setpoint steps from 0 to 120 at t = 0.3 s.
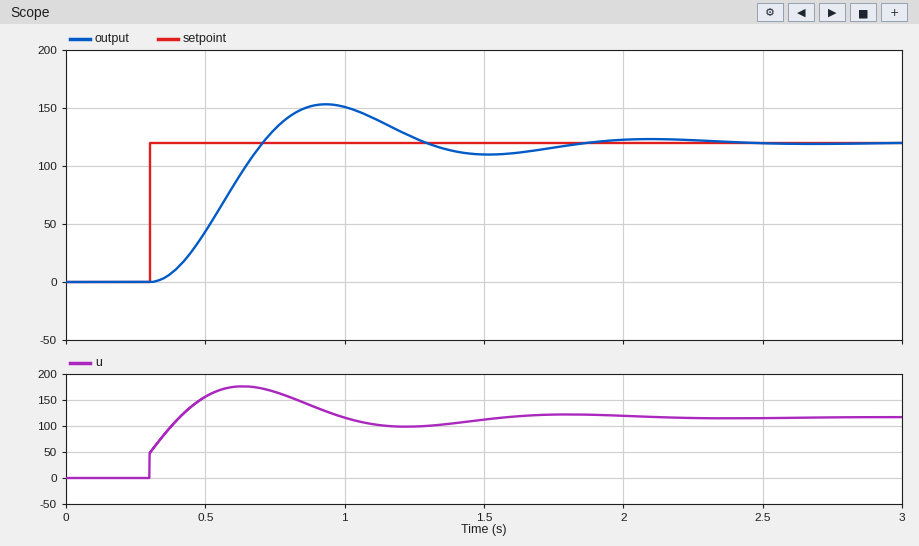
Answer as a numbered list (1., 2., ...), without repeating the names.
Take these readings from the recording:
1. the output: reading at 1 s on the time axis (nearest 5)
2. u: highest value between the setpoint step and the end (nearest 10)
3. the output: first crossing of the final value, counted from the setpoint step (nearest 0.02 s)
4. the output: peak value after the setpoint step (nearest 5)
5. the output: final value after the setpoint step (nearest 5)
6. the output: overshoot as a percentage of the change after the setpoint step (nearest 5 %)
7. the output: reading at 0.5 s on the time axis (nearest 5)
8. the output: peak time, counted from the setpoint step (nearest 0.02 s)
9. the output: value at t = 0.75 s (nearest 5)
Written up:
1. 150
2. 180
3. 0.40 s
4. 155
5. 120
6. 30 %
7. 45
8. 0.64 s
9. 130
